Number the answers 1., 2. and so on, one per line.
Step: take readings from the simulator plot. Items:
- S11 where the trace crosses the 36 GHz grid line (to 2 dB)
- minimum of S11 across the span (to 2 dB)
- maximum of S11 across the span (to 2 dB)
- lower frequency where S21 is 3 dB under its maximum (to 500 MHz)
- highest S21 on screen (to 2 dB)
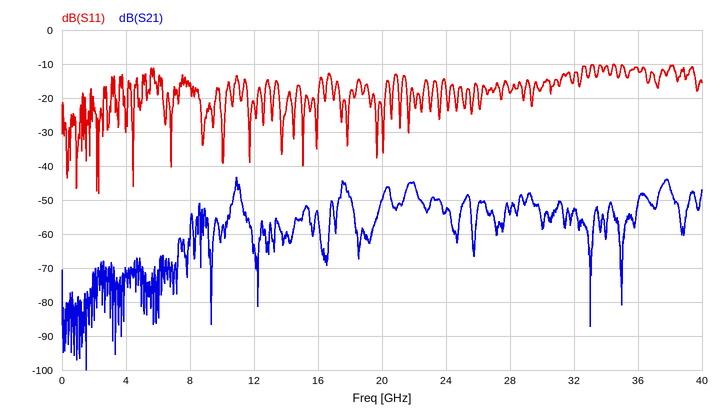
1. -12 dB
2. -48 dB
3. -10 dB
4. 11.0 GHz
5. -44 dB
